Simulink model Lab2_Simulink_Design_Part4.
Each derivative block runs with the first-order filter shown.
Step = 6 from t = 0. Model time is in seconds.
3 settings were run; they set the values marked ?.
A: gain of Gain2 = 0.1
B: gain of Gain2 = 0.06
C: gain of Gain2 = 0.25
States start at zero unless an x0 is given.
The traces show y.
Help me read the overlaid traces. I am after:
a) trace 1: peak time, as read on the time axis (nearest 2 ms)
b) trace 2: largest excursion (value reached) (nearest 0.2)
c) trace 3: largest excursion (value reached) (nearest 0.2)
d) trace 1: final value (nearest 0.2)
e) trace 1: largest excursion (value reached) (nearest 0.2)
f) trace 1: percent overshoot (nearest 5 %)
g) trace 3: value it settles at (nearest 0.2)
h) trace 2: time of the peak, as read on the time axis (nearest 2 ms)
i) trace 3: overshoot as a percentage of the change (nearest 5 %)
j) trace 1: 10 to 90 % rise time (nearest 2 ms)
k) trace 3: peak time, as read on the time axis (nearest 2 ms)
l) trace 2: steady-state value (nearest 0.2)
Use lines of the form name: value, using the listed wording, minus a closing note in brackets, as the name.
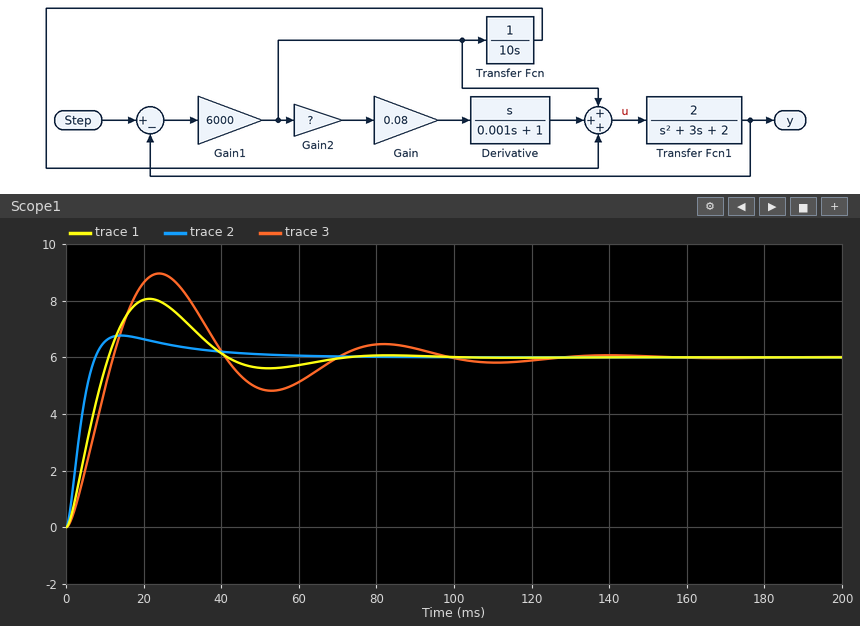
trace 1: peak time, as read on the time axis: 22 ms
trace 2: largest excursion (value reached): 6.8
trace 3: largest excursion (value reached): 9.0
trace 1: final value: 6.0
trace 1: largest excursion (value reached): 8.0
trace 1: percent overshoot: 35 %
trace 3: value it settles at: 6.0
trace 2: time of the peak, as read on the time axis: 14 ms
trace 3: overshoot as a percentage of the change: 50 %
trace 1: 10 to 90 % rise time: 8 ms
trace 3: peak time, as read on the time axis: 24 ms
trace 2: steady-state value: 6.0
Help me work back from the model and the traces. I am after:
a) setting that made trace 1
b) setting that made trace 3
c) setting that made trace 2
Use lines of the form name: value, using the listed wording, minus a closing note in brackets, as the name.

setting that made trace 1: A
setting that made trace 3: B
setting that made trace 2: C
